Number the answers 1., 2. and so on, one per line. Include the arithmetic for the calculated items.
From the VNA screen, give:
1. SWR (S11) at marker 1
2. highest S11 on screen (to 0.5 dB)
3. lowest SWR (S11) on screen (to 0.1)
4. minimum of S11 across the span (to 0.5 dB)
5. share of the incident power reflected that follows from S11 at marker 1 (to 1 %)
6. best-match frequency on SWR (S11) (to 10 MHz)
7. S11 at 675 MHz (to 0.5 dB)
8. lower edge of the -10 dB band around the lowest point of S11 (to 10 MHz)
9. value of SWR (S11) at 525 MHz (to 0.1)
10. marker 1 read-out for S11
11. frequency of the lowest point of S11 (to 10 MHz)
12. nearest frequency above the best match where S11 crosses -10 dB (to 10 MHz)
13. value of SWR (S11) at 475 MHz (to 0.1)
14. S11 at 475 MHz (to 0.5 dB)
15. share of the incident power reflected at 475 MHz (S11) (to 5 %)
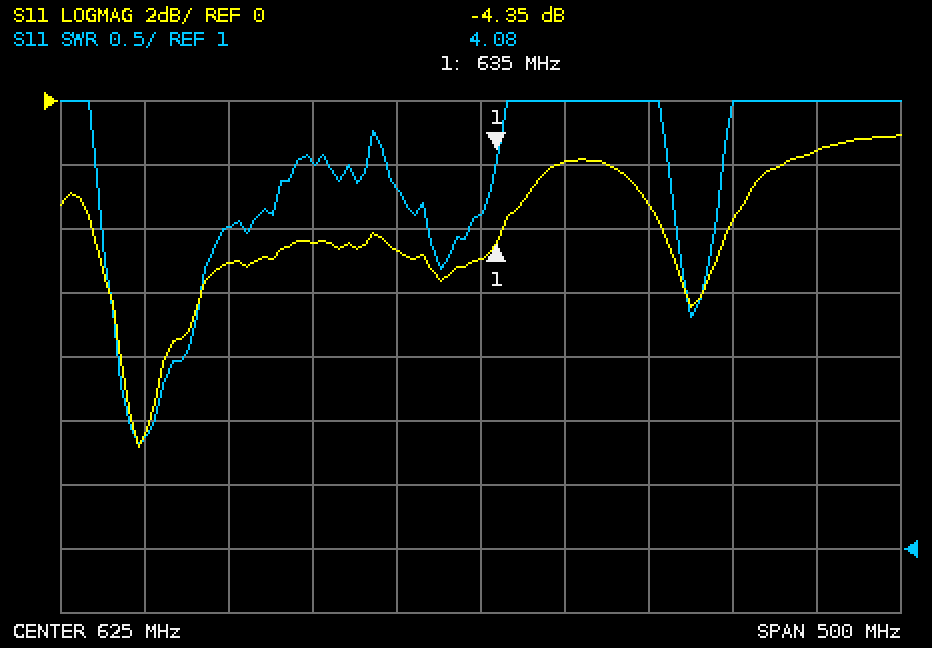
1. 4.08
2. -1.0 dB
3. 1.8
4. -11.0 dB
5. 10^(-4.35/10) ≈ 37 %
6. 420 MHz
7. -2.0 dB
8. 420 MHz
9. 4.0
10. -4.35 dB
11. 420 MHz
12. 430 MHz
13. 3.5
14. -5.0 dB
15. 10^(-5/10) ≈ 31.6 %, so 30 % to the nearest 5 %
